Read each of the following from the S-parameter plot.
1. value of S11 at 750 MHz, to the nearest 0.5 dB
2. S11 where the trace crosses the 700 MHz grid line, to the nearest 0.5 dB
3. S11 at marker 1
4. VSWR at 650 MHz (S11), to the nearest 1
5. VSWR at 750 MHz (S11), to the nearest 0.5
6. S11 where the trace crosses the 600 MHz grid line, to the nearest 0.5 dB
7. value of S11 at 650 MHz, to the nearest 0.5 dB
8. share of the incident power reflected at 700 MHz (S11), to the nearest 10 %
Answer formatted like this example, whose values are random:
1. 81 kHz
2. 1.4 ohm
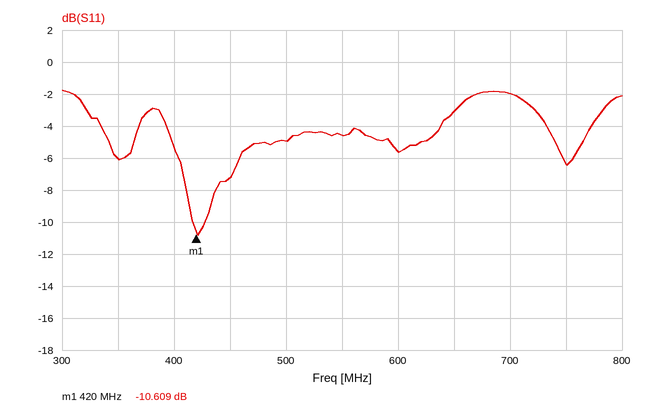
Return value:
1. -6.5 dB
2. -2.0 dB
3. -10.609 dB
4. 6
5. 3.0
6. -5.5 dB
7. -3.0 dB
8. 60 %
